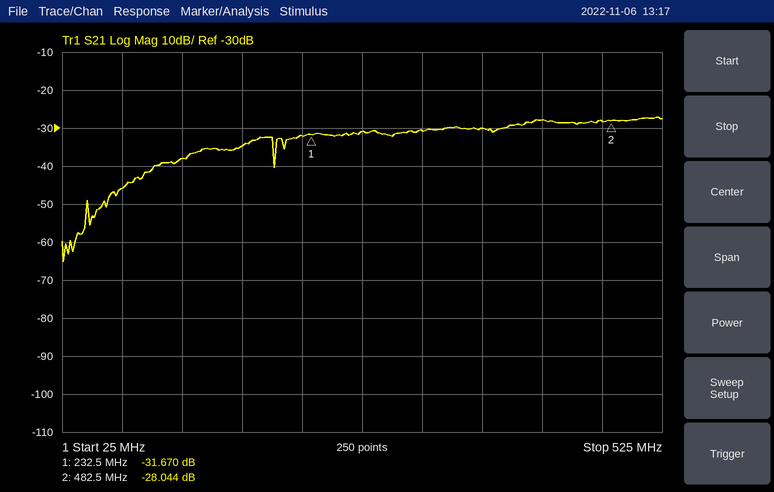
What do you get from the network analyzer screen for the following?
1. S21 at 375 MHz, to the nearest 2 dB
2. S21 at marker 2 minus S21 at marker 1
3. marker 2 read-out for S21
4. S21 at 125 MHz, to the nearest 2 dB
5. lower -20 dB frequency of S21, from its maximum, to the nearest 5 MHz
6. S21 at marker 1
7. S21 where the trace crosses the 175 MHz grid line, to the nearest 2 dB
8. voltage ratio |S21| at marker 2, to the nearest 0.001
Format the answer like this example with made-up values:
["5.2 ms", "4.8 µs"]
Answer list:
["-30 dB", "3.626 dB", "-28.044 dB", "-38 dB", "70 MHz", "-31.670 dB", "-34 dB", "0.040"]
